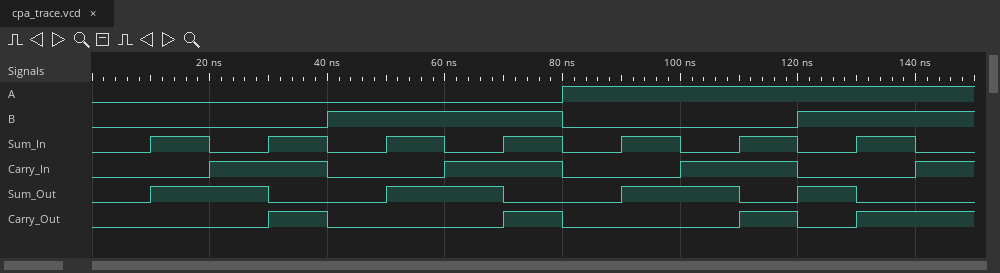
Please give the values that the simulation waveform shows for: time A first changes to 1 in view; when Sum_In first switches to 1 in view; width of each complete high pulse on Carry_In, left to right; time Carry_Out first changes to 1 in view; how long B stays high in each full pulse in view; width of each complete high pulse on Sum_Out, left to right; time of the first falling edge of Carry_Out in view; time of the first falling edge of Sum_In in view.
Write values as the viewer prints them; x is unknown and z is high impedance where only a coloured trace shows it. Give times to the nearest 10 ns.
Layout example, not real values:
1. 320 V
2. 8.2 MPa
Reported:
1. 80 ns
2. 10 ns
3. 20 ns, 20 ns, 20 ns
4. 30 ns
5. 40 ns
6. 20 ns, 20 ns, 20 ns, 10 ns
7. 40 ns
8. 20 ns
